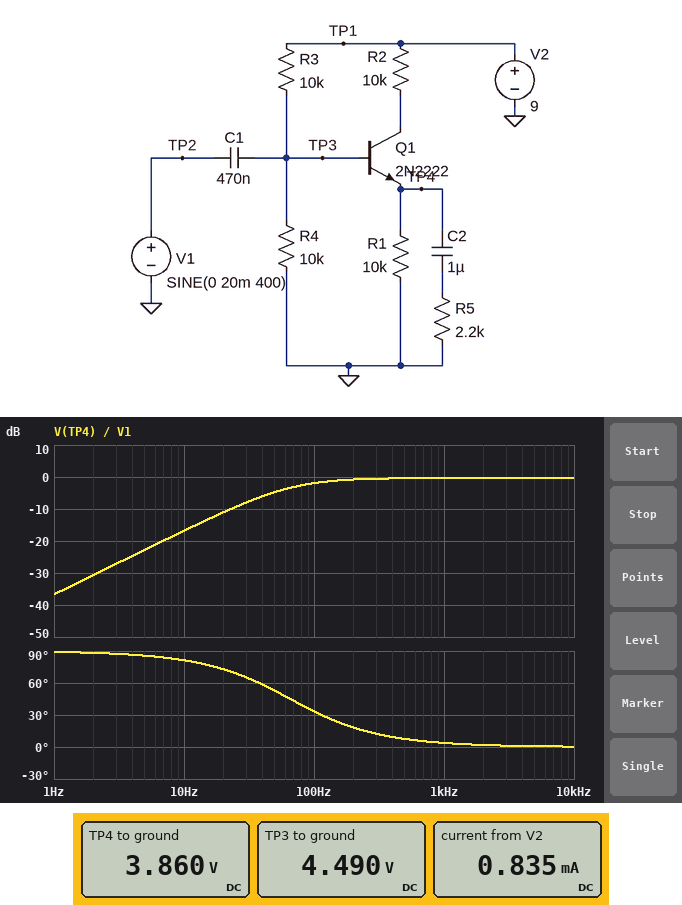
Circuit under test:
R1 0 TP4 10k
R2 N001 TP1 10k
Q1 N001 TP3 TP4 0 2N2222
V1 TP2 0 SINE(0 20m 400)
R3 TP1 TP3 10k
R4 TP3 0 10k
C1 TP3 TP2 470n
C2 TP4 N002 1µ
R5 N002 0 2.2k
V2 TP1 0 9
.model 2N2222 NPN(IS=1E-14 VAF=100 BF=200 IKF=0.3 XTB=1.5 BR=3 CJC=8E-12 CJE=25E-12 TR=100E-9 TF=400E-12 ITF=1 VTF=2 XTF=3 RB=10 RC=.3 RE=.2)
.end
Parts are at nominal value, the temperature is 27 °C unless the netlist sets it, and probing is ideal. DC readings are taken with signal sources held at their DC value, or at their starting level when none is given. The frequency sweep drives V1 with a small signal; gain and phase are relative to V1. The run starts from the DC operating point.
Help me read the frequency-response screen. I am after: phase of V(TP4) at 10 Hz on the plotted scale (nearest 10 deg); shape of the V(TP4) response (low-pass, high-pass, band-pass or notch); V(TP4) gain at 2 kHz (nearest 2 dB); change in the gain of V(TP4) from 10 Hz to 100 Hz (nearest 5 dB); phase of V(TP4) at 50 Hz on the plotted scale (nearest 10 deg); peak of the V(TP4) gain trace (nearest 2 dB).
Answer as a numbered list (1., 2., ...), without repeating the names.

1. 80 deg
2. high-pass
3. 0 dB
4. 15 dB
5. 50 deg
6. 0 dB
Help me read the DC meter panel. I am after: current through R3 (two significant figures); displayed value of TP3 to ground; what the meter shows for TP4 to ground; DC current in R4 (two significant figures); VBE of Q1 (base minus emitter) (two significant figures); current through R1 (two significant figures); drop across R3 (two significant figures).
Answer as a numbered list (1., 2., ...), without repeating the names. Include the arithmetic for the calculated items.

1. (9 V - 4.49 V) / 10 kΩ = 450 µA
2. 4.490 V
3. 3.860 V
4. (4.49 V) / 10 kΩ = 450 µA
5. 4.49 V - 3.86 V = 630 mV
6. (3.86 V) / 10 kΩ = 390 µA
7. 9 V - 4.49 V = 4.5 V
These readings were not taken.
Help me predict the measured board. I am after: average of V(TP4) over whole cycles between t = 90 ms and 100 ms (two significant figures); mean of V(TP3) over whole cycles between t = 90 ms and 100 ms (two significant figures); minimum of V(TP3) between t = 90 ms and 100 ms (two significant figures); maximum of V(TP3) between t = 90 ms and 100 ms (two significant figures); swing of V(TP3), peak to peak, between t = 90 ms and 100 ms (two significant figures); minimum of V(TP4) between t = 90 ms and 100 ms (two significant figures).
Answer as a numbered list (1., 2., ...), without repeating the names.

1. 3.9 V
2. 4.5 V
3. 4.5 V
4. 4.5 V
5. 39 mV
6. 3.8 V
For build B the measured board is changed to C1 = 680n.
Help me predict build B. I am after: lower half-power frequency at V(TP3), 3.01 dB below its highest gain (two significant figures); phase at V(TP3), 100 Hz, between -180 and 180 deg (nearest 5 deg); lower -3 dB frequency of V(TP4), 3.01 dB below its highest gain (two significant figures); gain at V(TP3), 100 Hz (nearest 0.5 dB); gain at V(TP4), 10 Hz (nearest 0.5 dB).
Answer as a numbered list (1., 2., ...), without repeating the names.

1. 47 Hz
2. 25 deg
3. 45 Hz
4. -1.0 dB
5. -13.5 dB
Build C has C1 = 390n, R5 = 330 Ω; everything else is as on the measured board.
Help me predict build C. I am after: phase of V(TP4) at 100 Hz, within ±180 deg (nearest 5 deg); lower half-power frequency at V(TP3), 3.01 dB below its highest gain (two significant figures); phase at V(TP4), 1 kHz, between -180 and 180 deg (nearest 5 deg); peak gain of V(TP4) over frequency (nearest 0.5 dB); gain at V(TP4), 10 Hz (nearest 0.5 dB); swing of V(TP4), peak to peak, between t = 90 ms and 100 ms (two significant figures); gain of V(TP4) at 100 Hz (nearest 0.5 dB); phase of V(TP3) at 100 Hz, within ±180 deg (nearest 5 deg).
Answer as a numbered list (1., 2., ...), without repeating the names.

1. 35 deg
2. 83 Hz
3. 0 deg
4. -1.0 dB
5. -18.5 dB
6. 35 mV
7. -2.5 dB
8. 40 deg
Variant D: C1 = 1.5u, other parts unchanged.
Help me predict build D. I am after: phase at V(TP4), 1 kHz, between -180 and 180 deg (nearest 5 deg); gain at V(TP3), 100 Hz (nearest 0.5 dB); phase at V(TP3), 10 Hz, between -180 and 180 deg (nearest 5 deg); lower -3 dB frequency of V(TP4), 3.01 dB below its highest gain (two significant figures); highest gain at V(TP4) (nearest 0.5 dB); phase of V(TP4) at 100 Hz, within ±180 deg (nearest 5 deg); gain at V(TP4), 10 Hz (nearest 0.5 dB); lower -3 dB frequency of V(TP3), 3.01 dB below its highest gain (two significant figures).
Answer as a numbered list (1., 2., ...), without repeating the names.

1. 0 deg
2. 0 dB
3. 65 deg
4. 20 Hz
5. -0.5 dB
6. 10 deg
7. -7.5 dB
8. 21 Hz
